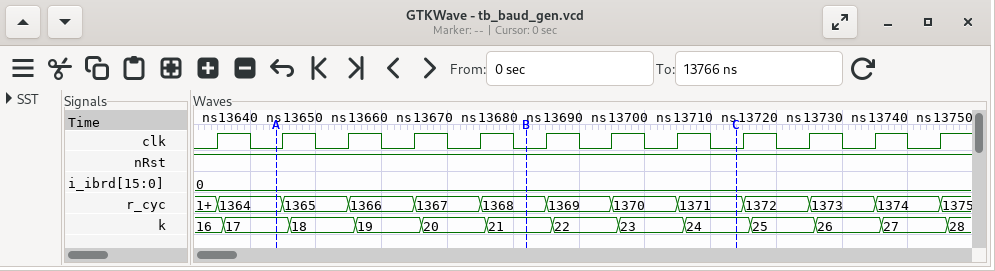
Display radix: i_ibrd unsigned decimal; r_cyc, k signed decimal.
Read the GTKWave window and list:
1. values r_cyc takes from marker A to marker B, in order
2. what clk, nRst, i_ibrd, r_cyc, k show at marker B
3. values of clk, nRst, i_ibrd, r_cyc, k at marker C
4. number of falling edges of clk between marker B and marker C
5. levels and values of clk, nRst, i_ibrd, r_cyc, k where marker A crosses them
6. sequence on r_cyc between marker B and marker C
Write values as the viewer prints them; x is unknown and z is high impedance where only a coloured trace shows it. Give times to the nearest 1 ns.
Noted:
1364, 1365, 1366, 1367, 1368
clk=0, nRst=1, i_ibrd=0, r_cyc=1368, k=21
clk=0, nRst=1, i_ibrd=0, r_cyc=1371, k=24
3
clk=0, nRst=1, i_ibrd=0, r_cyc=1364, k=17
1368, 1369, 1370, 1371
